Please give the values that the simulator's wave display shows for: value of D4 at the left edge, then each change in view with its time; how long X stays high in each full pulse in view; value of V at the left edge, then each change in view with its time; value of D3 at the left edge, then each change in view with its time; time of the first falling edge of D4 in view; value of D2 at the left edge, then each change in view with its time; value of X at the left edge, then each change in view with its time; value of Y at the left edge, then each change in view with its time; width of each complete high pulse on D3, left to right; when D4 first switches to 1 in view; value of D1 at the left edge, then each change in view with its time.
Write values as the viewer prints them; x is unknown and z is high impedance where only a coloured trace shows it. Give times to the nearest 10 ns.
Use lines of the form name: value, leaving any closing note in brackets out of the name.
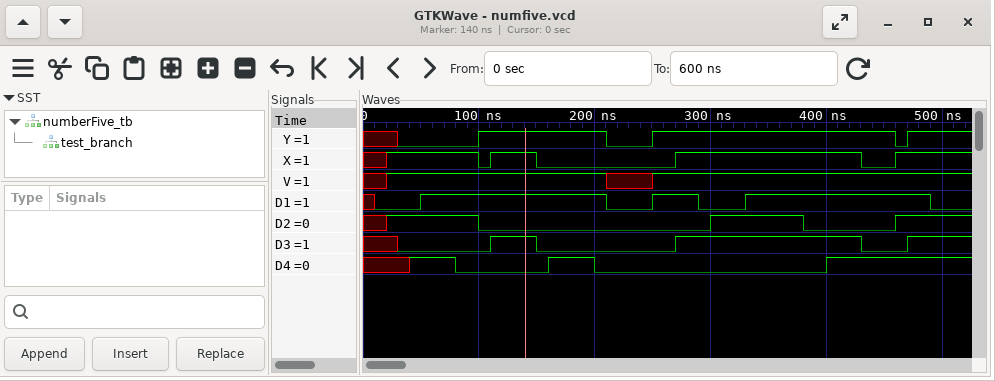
value of D4 at the left edge, then each change in view with its time: x, 1 at 40 ns, 0 at 80 ns, 1 at 160 ns, 0 at 200 ns, 1 at 400 ns
how long X stays high in each full pulse in view: 40 ns, 160 ns
value of V at the left edge, then each change in view with its time: x, 1 at 20 ns, x at 210 ns, 1 at 250 ns
value of D3 at the left edge, then each change in view with its time: x, 0 at 30 ns, 1 at 110 ns, 0 at 150 ns, 1 at 270 ns, 0 at 430 ns, 1 at 470 ns
time of the first falling edge of D4 in view: 80 ns
value of D2 at the left edge, then each change in view with its time: x, 1 at 20 ns, 0 at 100 ns, 1 at 300 ns, 0 at 380 ns, 1 at 460 ns
value of X at the left edge, then each change in view with its time: x, 1 at 20 ns, 0 at 100 ns, 1 at 110 ns, 0 at 150 ns, 1 at 270 ns, 0 at 430 ns, 1 at 460 ns
value of Y at the left edge, then each change in view with its time: x, 0 at 30 ns, 1 at 100 ns, 0 at 210 ns, 1 at 250 ns, 0 at 460 ns, 1 at 470 ns
width of each complete high pulse on D3, left to right: 40 ns, 160 ns
when D4 first switches to 1 in view: 40 ns
value of D1 at the left edge, then each change in view with its time: x, 0 at 10 ns, 1 at 50 ns, 0 at 210 ns, 1 at 250 ns, 0 at 290 ns, 1 at 330 ns, 0 at 490 ns
